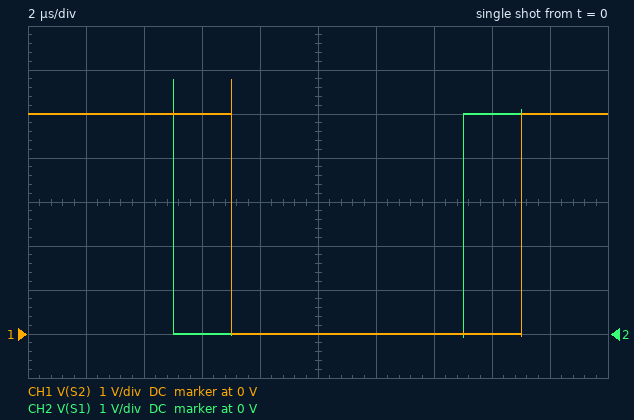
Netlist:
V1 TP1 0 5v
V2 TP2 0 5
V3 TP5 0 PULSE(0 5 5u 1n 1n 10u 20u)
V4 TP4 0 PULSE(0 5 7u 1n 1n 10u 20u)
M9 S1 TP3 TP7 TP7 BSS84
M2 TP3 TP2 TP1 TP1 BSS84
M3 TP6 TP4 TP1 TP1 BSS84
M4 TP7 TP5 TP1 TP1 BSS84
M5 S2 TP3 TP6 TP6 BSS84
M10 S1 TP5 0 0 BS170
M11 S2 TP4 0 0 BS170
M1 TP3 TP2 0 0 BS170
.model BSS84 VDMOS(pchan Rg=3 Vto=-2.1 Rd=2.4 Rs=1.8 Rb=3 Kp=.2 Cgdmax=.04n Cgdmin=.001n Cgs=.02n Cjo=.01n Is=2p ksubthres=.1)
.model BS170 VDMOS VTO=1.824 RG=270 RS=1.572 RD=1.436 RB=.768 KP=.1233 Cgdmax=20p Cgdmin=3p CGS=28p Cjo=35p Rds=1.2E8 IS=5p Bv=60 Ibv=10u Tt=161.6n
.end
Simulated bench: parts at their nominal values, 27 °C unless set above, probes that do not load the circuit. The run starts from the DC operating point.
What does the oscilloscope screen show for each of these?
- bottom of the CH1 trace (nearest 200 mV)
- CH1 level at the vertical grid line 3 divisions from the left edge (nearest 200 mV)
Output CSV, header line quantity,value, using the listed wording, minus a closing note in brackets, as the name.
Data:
quantity,value
bottom of the CH1 trace,0 V
CH1 level at the vertical grid line 3 divisions from the left edge,5.0 V
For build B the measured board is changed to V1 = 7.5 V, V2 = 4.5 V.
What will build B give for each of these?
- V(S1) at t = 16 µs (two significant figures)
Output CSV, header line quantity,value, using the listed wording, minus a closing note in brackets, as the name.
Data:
quantity,value
V(S1) at t = 16 µs,7.5 V
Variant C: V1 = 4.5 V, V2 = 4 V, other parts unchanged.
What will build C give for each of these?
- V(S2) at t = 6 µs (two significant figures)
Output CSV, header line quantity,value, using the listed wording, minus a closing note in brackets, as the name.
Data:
quantity,value
V(S2) at t = 6 µs,4.5 V
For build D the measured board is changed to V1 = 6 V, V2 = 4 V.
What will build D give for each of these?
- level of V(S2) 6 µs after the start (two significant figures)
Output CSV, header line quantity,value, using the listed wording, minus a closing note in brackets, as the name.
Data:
quantity,value
level of V(S2) 6 µs after the start,6.0 V
